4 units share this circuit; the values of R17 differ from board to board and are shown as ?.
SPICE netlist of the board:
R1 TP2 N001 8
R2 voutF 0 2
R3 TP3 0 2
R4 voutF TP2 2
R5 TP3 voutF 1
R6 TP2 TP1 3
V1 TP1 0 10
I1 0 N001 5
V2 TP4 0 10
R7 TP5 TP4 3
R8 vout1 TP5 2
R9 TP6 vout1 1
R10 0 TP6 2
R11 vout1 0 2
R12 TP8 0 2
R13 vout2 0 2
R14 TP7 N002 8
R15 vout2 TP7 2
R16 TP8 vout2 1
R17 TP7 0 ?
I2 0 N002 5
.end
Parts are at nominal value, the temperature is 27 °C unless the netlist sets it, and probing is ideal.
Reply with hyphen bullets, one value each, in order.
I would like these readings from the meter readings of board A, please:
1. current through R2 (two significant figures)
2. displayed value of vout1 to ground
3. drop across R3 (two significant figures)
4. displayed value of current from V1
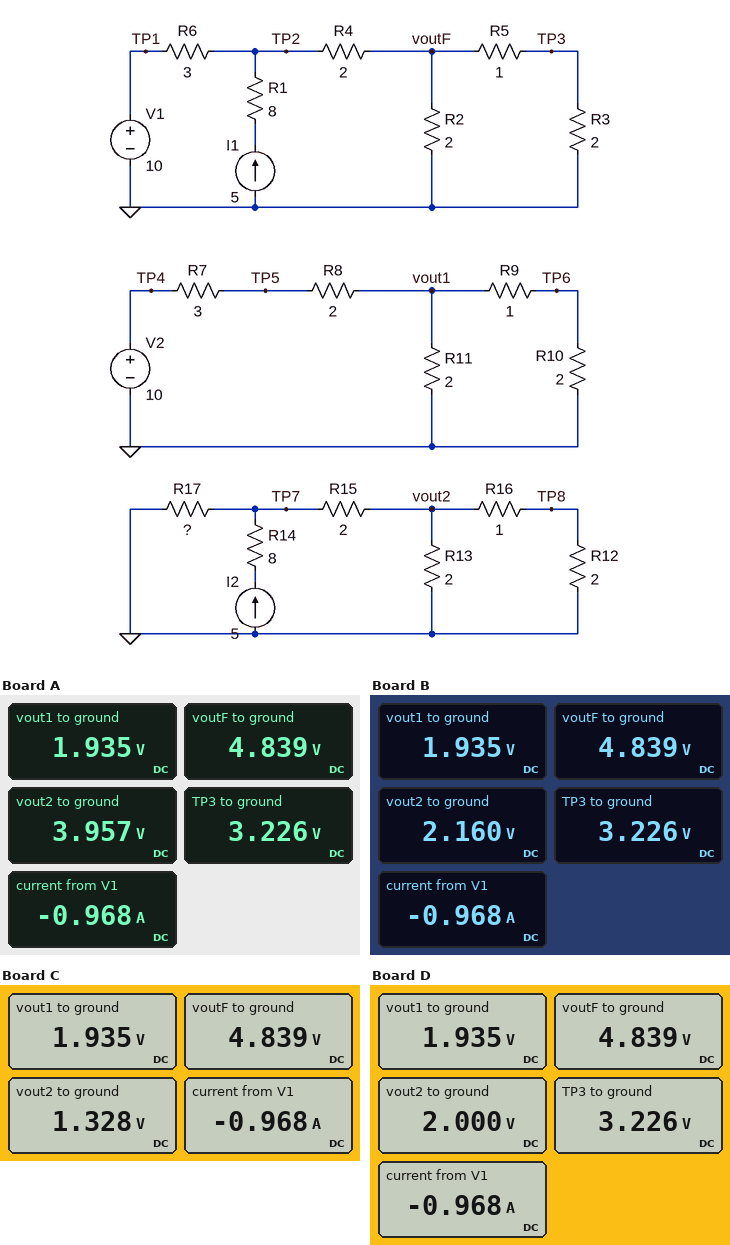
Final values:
- 2.4 A
- 1.935 V
- 3.2 V
- -0.968 A
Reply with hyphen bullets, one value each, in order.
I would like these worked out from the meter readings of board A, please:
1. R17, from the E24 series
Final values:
- 6.2 Ω
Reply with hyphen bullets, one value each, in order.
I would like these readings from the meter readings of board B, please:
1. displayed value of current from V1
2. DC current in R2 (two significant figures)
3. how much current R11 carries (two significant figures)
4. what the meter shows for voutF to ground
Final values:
- -0.968 A
- 2.4 A
- 970 mA
- 4.839 V
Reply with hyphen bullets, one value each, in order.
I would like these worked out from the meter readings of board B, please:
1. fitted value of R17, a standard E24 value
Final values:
- 1.8 Ω
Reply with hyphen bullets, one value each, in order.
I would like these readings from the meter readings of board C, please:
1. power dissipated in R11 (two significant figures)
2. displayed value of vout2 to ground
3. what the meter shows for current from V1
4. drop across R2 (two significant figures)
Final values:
- 1.9 W
- 1.328 V
- -0.968 A
- 4.8 V
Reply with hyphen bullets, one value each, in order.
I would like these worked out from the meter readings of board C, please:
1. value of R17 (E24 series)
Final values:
- 0.91 Ω
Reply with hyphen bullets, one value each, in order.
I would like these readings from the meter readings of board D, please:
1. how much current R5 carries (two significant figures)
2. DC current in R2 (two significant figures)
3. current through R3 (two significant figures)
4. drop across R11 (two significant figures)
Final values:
- 1.6 A
- 2.4 A
- 1.6 A
- 1.9 V
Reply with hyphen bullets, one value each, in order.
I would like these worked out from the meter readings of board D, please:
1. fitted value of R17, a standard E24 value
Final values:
- 1.6 Ω
